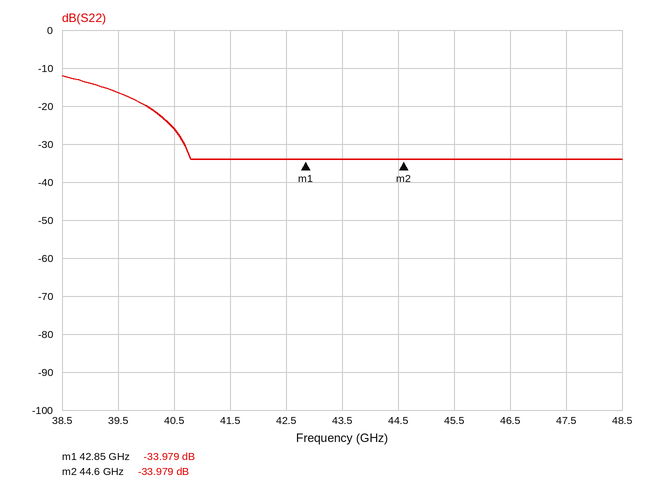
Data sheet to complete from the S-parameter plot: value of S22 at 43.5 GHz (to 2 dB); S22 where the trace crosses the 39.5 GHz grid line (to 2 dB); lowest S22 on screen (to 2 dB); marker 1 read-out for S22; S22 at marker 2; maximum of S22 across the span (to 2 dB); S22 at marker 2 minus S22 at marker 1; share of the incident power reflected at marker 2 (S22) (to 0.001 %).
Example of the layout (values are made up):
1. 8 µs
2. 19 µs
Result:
1. -34 dB
2. -16 dB
3. -34 dB
4. -33.979 dB
5. -33.979 dB
6. -12 dB
7. 0.000 dB
8. 0.040 %
